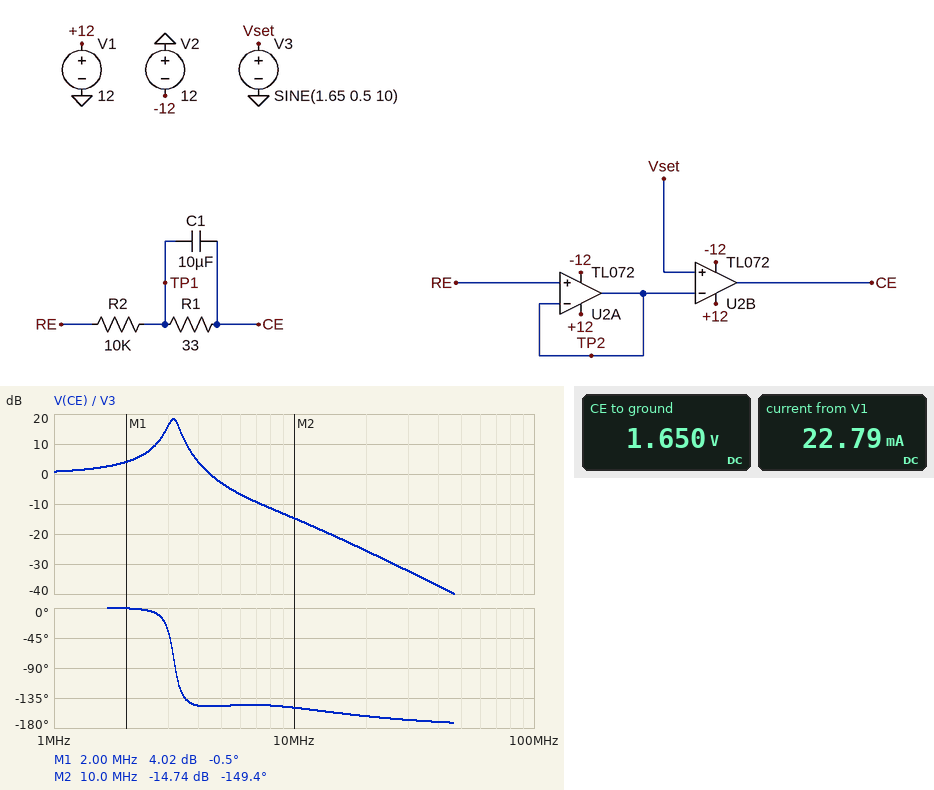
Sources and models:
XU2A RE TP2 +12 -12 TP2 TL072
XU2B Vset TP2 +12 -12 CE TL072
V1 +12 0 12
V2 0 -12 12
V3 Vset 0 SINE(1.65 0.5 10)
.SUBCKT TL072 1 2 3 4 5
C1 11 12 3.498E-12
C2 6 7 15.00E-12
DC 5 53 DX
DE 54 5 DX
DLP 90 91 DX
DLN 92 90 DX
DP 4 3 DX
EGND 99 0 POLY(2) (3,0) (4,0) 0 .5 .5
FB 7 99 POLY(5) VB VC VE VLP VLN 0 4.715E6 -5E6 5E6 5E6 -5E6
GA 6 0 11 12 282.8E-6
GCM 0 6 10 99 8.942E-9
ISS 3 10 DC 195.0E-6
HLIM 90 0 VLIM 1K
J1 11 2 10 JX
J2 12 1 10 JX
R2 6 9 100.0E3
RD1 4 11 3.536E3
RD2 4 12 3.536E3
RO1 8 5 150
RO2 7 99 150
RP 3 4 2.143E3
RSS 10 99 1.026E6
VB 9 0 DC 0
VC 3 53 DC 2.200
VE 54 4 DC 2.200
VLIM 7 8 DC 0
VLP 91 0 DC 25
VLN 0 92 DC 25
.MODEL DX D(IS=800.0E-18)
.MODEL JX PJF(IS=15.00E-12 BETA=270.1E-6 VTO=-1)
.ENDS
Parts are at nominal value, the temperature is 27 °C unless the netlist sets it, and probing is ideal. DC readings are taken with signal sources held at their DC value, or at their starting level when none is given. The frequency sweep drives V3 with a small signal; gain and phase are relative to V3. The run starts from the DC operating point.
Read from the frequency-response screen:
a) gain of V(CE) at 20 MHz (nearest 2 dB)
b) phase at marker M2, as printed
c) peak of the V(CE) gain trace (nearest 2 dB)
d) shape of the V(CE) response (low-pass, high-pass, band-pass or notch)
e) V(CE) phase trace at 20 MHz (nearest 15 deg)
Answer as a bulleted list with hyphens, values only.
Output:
- -26 dB
- -149.4 deg
- 18 dB
- low-pass
- -165 deg
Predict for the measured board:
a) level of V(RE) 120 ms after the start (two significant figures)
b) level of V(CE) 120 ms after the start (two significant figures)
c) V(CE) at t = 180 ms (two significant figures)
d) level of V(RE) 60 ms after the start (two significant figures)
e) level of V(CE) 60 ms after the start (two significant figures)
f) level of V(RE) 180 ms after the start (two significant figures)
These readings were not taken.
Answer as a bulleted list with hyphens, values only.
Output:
- 2.1 V
- 2.1 V
- 1.2 V
- 1.4 V
- 1.4 V
- 1.2 V
